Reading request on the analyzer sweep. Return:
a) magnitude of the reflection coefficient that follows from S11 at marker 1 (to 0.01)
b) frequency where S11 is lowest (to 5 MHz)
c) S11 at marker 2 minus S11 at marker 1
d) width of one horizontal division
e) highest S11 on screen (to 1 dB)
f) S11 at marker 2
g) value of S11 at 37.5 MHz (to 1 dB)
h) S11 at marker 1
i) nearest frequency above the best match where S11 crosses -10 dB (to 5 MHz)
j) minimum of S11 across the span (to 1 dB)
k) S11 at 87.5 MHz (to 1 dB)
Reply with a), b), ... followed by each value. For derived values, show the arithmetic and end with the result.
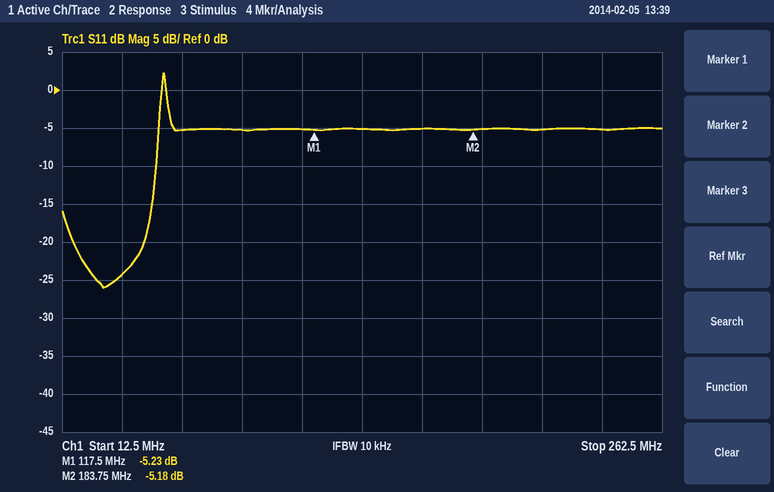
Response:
a) 10^(-5.23/20) ≈ 0.55
b) 30 MHz
c) -5.18 − (-5.23) = 0.05 dB
d) 25 MHz
e) 2 dB
f) -5.18 dB
g) -24 dB
h) -5.23 dB
i) 50 MHz
j) -26 dB
k) -5 dB
